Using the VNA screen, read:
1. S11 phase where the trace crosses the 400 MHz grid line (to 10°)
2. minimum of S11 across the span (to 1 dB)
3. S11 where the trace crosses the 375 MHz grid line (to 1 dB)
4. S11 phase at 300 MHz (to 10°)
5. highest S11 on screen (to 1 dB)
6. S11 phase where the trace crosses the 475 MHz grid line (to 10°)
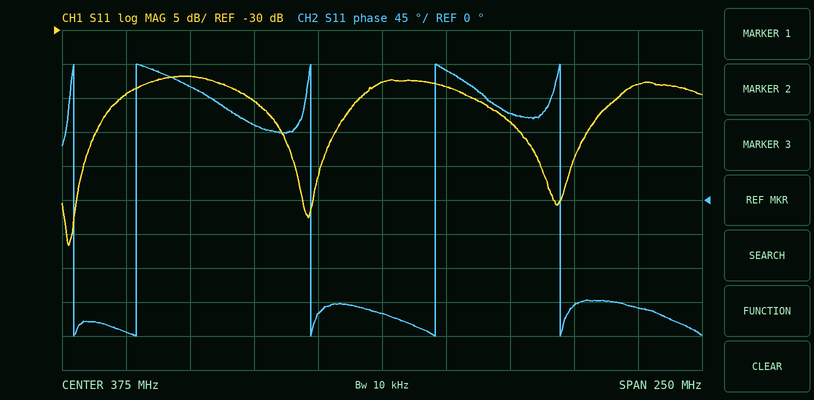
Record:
170°
-62 dB
-38 dB
150°
-37 dB
-140°
